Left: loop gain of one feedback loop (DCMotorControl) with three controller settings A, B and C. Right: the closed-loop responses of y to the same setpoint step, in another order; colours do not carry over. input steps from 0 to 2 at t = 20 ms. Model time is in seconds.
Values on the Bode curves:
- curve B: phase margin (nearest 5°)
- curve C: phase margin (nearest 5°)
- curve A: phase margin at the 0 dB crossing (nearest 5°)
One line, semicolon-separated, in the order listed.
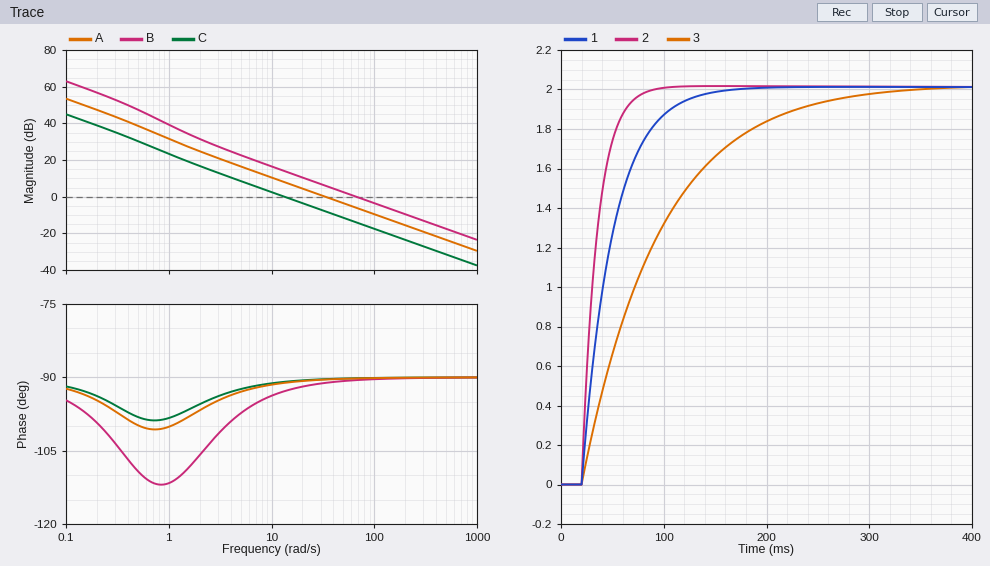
90°; 90°; 90°
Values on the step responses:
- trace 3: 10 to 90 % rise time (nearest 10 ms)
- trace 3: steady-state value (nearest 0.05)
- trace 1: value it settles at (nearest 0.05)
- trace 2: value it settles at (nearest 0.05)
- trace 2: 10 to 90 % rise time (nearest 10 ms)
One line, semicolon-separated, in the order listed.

160 ms; 2.00; 2.00; 2.00; 30 ms
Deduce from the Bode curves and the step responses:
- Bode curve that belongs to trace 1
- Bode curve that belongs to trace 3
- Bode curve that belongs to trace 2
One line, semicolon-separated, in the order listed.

A; C; B
